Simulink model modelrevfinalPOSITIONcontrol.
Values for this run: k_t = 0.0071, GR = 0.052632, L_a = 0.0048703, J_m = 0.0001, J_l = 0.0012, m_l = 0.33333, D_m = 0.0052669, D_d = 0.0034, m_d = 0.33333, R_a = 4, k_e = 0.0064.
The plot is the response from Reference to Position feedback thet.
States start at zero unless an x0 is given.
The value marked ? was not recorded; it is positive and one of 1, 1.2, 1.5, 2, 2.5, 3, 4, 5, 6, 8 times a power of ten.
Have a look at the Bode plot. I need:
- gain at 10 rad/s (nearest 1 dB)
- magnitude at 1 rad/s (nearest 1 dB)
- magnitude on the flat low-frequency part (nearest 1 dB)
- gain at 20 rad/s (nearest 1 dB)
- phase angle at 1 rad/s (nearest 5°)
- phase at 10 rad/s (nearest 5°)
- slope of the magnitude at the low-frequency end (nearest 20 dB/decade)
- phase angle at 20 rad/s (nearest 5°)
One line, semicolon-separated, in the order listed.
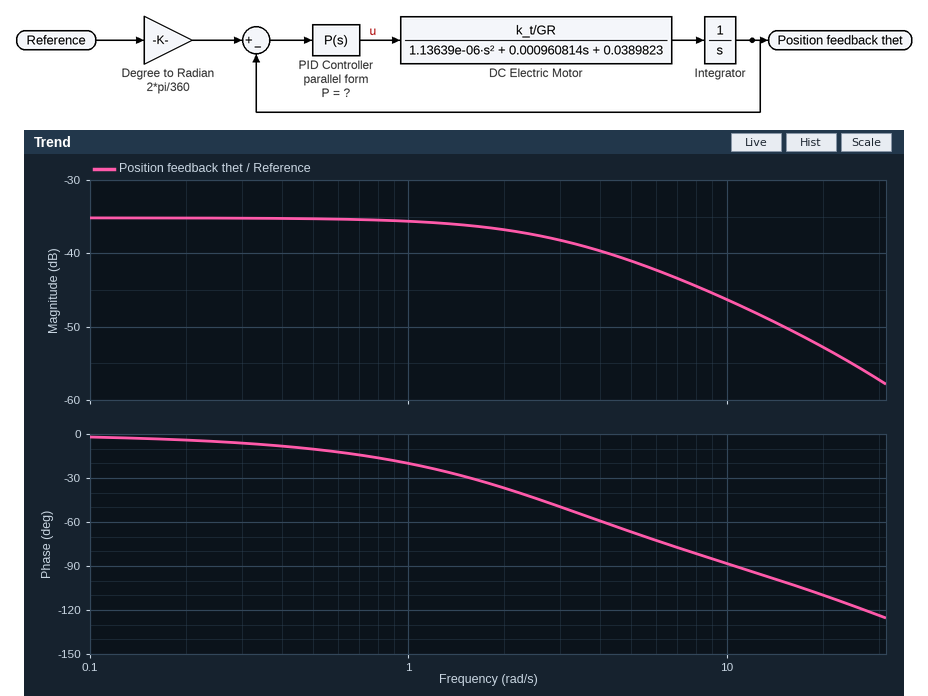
-46 dB; -36 dB; -35 dB; -53 dB; -20°; -90°; 0 dB/decade; -110°
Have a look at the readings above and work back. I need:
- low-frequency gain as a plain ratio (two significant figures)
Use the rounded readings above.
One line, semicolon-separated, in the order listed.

0.018
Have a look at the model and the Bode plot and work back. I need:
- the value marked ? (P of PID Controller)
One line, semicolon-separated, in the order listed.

0.8
